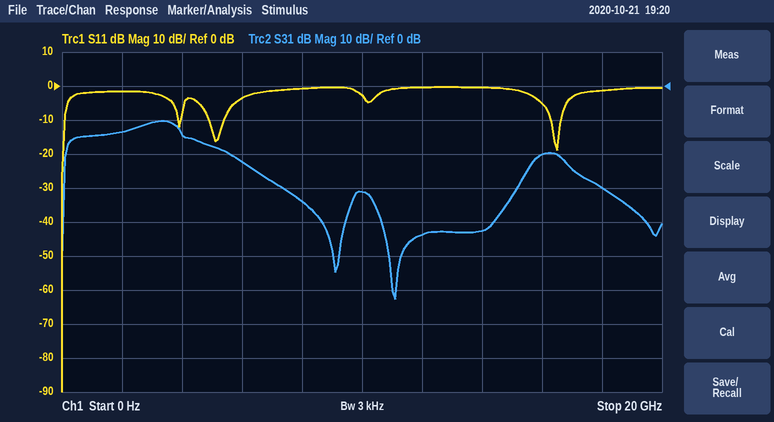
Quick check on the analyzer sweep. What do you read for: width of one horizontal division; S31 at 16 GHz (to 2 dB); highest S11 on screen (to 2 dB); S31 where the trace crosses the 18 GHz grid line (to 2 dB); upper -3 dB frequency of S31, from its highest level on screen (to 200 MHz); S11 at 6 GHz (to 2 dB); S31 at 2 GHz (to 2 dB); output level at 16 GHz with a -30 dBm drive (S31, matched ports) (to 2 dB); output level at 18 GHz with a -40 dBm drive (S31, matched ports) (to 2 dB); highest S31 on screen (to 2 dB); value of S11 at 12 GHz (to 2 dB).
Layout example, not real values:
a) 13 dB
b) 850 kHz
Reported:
a) 2 GHz
b) -20 dB
c) 0 dB
d) -30 dB
e) 4.0 GHz
f) -4 dB
g) -14 dB
h) -50 dBm
i) -70 dBm
j) -10 dB
k) 0 dB
